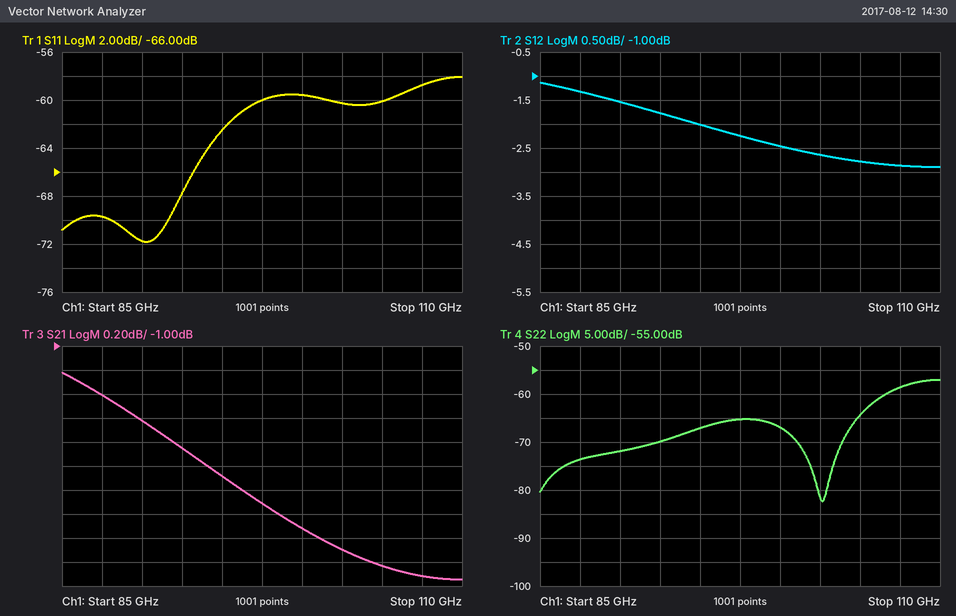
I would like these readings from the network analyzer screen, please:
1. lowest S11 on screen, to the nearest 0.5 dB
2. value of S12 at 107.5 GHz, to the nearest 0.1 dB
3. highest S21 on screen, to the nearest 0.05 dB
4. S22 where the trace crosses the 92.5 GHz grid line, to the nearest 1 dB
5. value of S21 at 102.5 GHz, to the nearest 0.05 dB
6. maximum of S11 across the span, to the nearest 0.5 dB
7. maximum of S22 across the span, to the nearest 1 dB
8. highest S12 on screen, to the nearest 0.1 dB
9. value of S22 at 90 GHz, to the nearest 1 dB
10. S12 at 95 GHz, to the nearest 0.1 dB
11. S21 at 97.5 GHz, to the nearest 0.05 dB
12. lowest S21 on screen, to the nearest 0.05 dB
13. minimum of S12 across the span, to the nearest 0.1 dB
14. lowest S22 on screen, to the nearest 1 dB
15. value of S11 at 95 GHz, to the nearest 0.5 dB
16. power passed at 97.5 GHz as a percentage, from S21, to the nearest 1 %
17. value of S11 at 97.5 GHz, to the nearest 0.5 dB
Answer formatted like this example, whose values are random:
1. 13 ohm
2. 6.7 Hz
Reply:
1. -72.0 dB
2. -2.9 dB
3. -1.20 dB
4. -70 dB
5. -2.70 dB
6. -58.0 dB
7. -57 dB
8. -1.1 dB
9. -72 dB
10. -2.0 dB
11. -2.30 dB
12. -2.95 dB
13. -2.9 dB
14. -82 dB
15. -62.5 dB
16. 59 %
17. -60.0 dB
